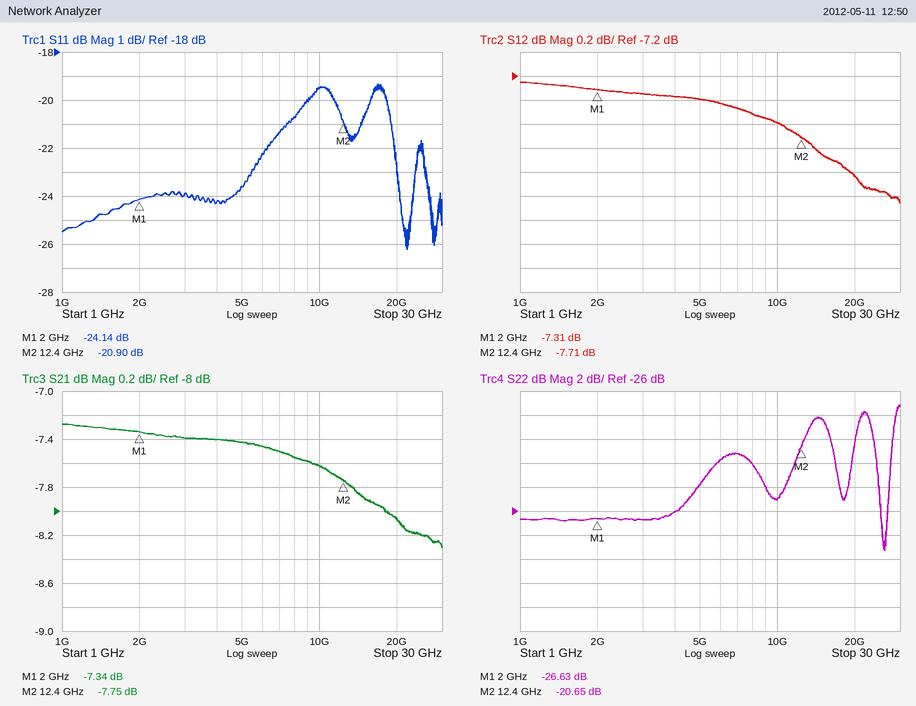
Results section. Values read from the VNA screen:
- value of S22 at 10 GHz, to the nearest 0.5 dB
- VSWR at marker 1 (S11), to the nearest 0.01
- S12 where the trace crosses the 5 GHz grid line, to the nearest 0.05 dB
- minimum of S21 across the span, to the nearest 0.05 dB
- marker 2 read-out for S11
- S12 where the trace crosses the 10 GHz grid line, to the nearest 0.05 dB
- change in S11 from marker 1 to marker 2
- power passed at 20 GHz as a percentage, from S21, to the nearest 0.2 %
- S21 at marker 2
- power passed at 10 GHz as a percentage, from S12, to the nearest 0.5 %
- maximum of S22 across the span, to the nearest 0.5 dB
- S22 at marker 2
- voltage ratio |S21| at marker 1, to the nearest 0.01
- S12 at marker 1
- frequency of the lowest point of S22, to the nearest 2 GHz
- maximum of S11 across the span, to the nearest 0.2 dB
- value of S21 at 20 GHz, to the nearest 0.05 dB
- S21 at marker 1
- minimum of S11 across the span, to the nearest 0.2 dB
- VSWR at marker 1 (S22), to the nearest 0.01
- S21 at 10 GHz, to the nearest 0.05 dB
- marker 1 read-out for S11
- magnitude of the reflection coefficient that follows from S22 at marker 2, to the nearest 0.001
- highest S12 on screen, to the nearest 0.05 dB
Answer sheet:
-25.0 dB
1.13
-7.40 dB
-8.30 dB
-20.90 dB
-7.60 dB
3.24 dB
15.6 %
-7.75 dB
17.5 %
-17.0 dB
-20.65 dB
0.43
-7.31 dB
26 GHz
-19.4 dB
-8.05 dB
-7.34 dB
-26.2 dB
1.10
-7.60 dB
-24.14 dB
0.093
-7.25 dB
